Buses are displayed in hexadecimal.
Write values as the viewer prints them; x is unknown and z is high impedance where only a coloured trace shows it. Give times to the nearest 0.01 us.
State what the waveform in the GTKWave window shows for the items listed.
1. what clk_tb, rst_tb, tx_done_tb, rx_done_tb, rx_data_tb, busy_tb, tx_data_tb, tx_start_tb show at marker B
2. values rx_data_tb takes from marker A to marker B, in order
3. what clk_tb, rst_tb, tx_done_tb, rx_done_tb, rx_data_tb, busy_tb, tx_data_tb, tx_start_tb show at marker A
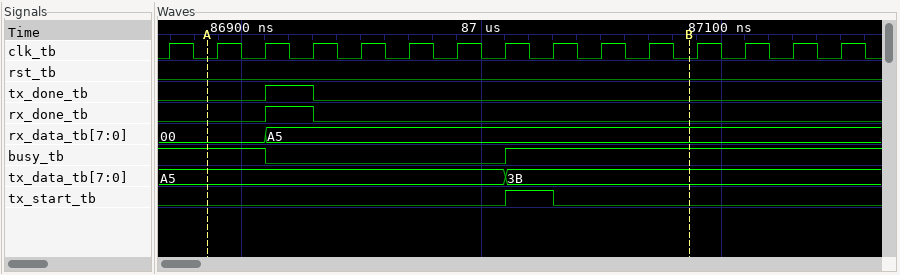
clk_tb=0, rst_tb=0, tx_done_tb=0, rx_done_tb=0, rx_data_tb=A5, busy_tb=1, tx_data_tb=3B, tx_start_tb=0
00, A5
clk_tb=0, rst_tb=0, tx_done_tb=0, rx_done_tb=0, rx_data_tb=00, busy_tb=1, tx_data_tb=A5, tx_start_tb=0
